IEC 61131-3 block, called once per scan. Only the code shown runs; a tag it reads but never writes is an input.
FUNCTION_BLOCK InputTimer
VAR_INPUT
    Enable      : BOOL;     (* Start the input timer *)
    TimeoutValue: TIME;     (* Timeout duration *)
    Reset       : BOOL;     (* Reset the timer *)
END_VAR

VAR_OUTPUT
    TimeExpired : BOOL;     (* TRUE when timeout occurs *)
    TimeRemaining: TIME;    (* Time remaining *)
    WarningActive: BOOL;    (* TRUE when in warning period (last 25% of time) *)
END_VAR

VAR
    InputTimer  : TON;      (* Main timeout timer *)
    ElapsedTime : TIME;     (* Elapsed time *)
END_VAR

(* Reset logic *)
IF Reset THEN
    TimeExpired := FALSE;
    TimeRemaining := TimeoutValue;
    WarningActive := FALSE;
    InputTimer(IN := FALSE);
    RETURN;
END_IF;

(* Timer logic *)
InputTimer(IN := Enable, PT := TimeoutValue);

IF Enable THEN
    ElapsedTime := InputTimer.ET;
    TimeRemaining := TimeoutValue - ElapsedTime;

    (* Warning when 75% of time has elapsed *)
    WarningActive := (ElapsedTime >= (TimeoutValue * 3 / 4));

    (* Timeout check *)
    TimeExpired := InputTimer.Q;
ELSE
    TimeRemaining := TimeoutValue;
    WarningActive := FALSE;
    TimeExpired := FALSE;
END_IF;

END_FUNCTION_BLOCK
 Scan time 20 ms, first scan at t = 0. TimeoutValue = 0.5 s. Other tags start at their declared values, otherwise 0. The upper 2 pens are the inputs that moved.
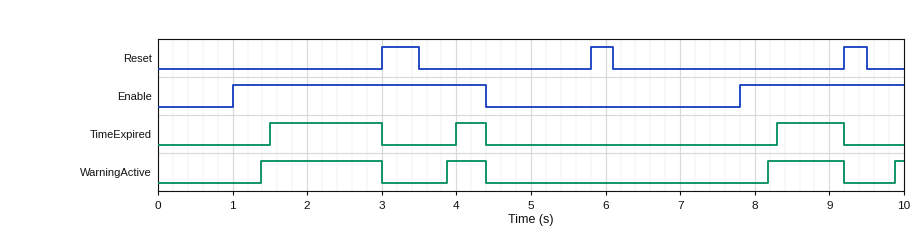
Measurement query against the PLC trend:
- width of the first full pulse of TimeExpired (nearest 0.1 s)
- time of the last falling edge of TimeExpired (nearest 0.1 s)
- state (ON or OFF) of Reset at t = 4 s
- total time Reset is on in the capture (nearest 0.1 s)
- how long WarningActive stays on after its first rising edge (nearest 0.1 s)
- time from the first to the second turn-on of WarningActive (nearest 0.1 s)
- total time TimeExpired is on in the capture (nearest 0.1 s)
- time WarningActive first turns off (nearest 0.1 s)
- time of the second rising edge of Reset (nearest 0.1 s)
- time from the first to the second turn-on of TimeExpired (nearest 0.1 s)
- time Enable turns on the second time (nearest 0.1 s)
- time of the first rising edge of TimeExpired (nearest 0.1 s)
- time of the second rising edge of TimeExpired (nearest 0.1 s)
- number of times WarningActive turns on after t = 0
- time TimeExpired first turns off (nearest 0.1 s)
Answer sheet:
1.5 s
9.2 s
OFF
1.1 s
1.6 s
2.5 s
2.8 s
3.0 s
5.8 s
2.5 s
7.8 s
1.5 s
4.0 s
4
3.0 s
